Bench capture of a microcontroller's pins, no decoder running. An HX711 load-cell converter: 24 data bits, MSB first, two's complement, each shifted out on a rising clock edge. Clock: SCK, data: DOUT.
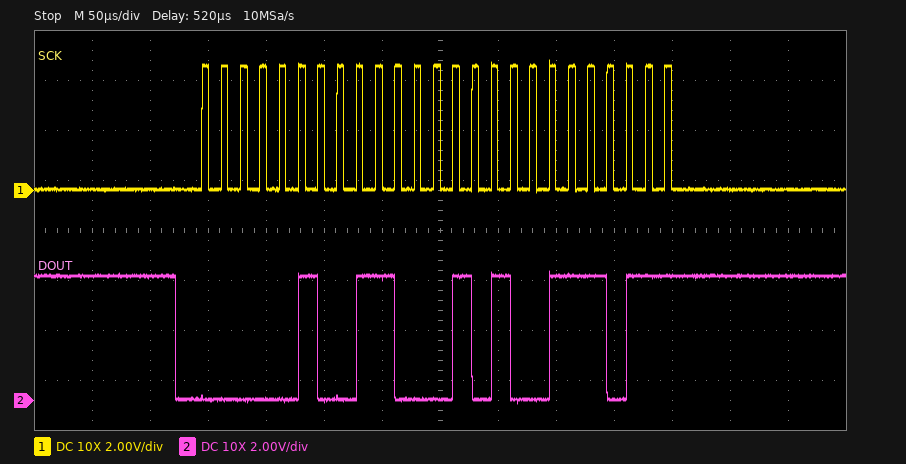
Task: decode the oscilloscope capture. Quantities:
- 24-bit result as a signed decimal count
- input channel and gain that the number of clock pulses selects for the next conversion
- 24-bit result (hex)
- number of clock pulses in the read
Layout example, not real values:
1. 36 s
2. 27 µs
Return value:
1. 312635
2. channel A, gain 128
3. 0x04C53B
4. 25
